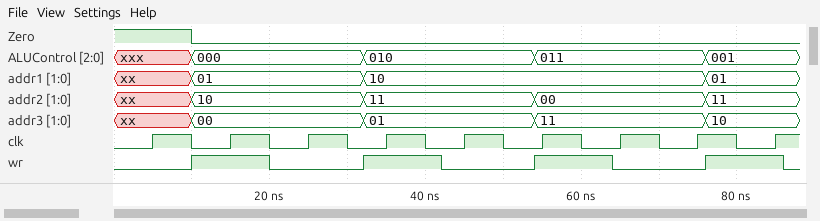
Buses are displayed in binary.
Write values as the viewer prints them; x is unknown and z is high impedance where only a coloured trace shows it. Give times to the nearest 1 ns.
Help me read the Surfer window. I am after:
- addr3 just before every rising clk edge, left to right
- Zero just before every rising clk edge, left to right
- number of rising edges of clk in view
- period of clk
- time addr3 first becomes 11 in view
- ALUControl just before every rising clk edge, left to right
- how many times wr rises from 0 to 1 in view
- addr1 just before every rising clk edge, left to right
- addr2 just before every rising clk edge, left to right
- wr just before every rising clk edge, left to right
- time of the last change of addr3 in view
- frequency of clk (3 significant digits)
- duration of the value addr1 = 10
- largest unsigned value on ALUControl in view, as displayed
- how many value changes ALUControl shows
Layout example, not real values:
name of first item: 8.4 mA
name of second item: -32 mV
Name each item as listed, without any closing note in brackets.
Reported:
addr3 just before every rising clk edge, left to right: xx, 00, 00, 01, 01, 11, 11, 11, 10
Zero just before every rising clk edge, left to right: 1 0 0 0 0 0 0 0 0
number of rising edges of clk in view: 9
period of clk: 10 ns
time addr3 first becomes 11 in view: 54 ns
ALUControl just before every rising clk edge, left to right: xxx, 000, 000, 010, 010, 011, 011, 011, 001
how many times wr rises from 0 to 1 in view: 4
addr1 just before every rising clk edge, left to right: xx, 01, 01, 10, 10, 10, 10, 10, 01
addr2 just before every rising clk edge, left to right: xx, 10, 10, 11, 11, 00, 00, 00, 11
wr just before every rising clk edge, left to right: 0 1 0 1 0 1 0 0 1
time of the last change of addr3 in view: 76 ns
frequency of clk: 100 MHz
duration of the value addr1 = 10: 44 ns
largest unsigned value on ALUControl in view, as displayed: 011
how many value changes ALUControl shows: 4
